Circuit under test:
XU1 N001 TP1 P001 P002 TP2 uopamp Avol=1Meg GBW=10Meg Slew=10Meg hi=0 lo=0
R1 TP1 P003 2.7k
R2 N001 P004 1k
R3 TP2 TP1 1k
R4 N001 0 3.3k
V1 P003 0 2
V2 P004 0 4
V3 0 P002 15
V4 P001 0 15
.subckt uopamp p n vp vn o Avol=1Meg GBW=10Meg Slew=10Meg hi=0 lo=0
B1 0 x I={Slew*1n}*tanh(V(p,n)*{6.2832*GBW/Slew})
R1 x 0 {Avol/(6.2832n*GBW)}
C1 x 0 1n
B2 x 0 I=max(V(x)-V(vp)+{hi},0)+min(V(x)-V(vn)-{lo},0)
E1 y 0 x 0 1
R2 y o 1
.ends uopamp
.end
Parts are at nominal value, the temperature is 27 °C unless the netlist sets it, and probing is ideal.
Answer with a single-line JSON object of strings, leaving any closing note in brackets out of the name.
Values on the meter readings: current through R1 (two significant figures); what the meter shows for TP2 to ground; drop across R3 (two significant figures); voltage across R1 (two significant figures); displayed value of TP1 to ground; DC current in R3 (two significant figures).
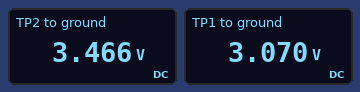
{"current through R1": "400 µA", "what the meter shows for TP2 to ground": "3.466 V", "drop across R3": "400 mV", "voltage across R1": "1.1 V", "displayed value of TP1 to ground": "3.070 V", "DC current in R3": "400 µA"}
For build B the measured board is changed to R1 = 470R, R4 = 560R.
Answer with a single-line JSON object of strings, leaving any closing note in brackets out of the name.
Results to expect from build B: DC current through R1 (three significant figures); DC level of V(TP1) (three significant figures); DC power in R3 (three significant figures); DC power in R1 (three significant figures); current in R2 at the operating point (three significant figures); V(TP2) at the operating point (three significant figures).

{"DC current through R1": "1.20 mA", "DC level of V(TP1)": "1.44 V", "DC power in R3": "1.44 mW", "DC power in R1": "677 µW", "current in R2 at the operating point": "2.56 mA", "V(TP2) at the operating point": "236 mV"}
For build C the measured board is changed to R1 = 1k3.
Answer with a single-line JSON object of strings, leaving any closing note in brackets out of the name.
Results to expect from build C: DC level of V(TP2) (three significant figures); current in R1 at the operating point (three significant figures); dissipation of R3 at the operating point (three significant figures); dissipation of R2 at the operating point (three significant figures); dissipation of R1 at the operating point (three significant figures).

{"DC level of V(TP2)": "3.89 V", "current in R1 at the operating point": "823 µA", "dissipation of R3 at the operating point": "677 µW", "dissipation of R2 at the operating point": "865 µW", "dissipation of R1 at the operating point": "880 µW"}
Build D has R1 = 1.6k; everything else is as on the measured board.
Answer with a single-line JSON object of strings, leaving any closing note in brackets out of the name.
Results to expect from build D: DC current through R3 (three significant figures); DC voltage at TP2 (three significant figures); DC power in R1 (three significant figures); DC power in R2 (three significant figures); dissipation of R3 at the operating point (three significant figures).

{"DC current through R3": "669 µA", "DC voltage at TP2": "3.74 V", "DC power in R1": "715 µW", "DC power in R2": "865 µW", "dissipation of R3 at the operating point": "447 µW"}
